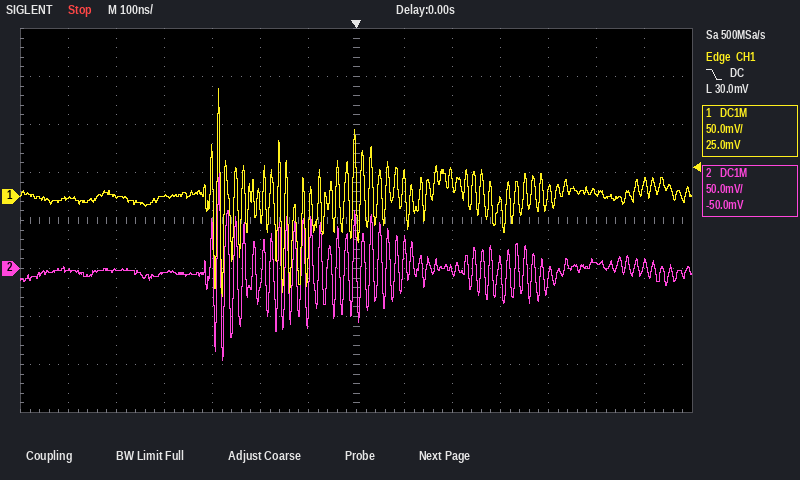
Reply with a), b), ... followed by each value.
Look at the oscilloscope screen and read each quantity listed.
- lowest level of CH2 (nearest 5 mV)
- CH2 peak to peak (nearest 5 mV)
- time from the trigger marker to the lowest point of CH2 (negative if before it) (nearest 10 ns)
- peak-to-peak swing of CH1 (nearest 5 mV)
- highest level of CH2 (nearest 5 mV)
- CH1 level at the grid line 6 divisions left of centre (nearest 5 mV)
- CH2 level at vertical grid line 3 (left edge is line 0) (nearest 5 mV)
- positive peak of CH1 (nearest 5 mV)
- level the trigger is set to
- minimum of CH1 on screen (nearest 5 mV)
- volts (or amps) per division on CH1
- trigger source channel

a) -95 mV
b) 195 mV
c) -280 ns
d) 215 mV
e) 100 mV
f) 0 mV
g) -5 mV
h) 110 mV
i) 30.0 mV
j) -105 mV
k) 50 mV
l) CH1
